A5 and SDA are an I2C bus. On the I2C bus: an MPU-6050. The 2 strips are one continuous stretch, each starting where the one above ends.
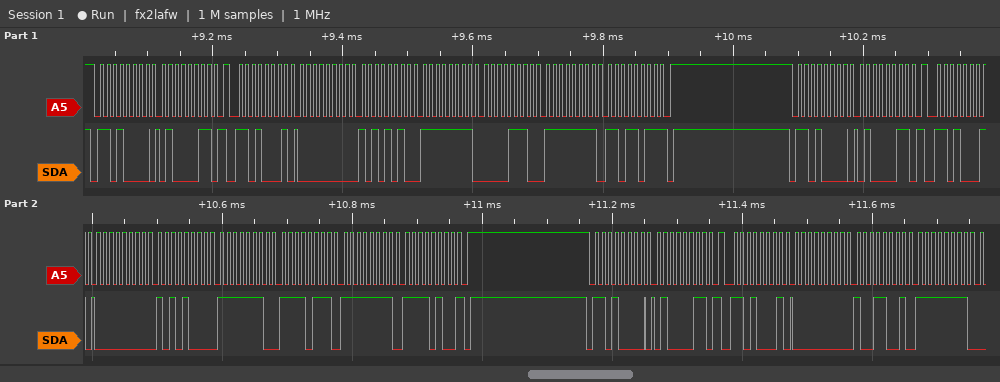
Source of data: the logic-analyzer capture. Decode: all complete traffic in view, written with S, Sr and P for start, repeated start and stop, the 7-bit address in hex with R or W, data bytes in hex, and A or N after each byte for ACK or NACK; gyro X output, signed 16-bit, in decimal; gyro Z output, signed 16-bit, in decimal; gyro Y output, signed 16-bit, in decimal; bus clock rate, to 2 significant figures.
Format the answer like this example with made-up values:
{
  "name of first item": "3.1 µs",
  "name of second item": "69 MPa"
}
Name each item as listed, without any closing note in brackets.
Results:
{
  "all complete traffic in view, written with S, Sr and P for start, repeated start and stop, the 7-bit address in hex with R or W, data bytes in hex, and A or N after each byte for ACK or NACK": "S 68W A 43 A Sr 68R A 00 A AA A FF A 0E A FF A DB N P S 68W A 43 A Sr 68R A 00 A A8 A FE A F7 A FF A F4 N P S 68W A 43 A Sr 68R A 00 A 99 A FF A",
  "gyro X output, signed 16-bit, in decimal": "170",
  "gyro Z output, signed 16-bit, in decimal": "-37",
  "gyro Y output, signed 16-bit, in decimal": "-242",
  "bus clock rate, to 2 significant figures": "100 kHz"
}
